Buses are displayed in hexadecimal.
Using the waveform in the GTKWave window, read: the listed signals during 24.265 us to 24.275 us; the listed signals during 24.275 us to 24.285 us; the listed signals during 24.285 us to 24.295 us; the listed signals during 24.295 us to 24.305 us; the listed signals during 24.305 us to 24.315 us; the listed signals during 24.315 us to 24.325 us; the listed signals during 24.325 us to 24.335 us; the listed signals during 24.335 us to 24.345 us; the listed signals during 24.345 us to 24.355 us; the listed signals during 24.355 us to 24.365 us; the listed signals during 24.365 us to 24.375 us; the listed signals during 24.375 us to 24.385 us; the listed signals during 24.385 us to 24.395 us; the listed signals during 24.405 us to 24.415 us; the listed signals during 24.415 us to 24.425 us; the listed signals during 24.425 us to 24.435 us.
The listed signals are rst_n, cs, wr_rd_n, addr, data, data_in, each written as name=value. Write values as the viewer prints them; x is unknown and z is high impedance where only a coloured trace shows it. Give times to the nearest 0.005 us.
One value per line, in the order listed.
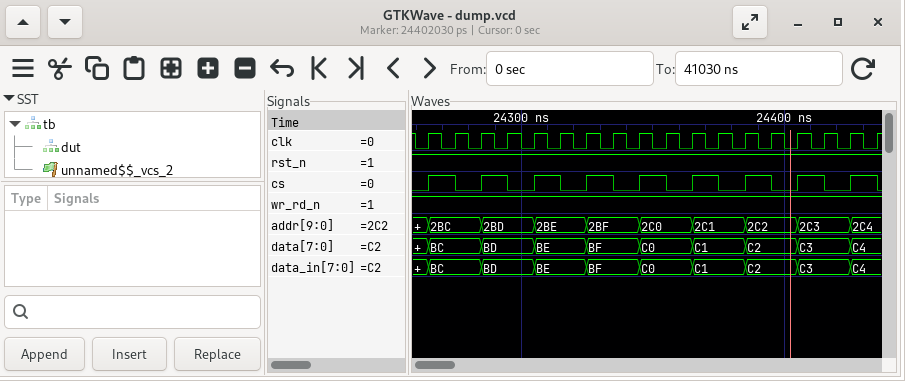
rst_n=1, cs=1, wr_rd_n=1, addr=2BC, data=BC, data_in=BC
rst_n=1, cs=0, wr_rd_n=1, addr=2BC, data=BC, data_in=BC
rst_n=1, cs=1, wr_rd_n=1, addr=2BD, data=BD, data_in=BD
rst_n=1, cs=0, wr_rd_n=1, addr=2BD, data=BD, data_in=BD
rst_n=1, cs=1, wr_rd_n=1, addr=2BE, data=BE, data_in=BE
rst_n=1, cs=0, wr_rd_n=1, addr=2BE, data=BE, data_in=BE
rst_n=1, cs=1, wr_rd_n=1, addr=2BF, data=BF, data_in=BF
rst_n=1, cs=0, wr_rd_n=1, addr=2BF, data=BF, data_in=BF
rst_n=1, cs=1, wr_rd_n=1, addr=2C0, data=C0, data_in=C0
rst_n=1, cs=0, wr_rd_n=1, addr=2C0, data=C0, data_in=C0
rst_n=1, cs=1, wr_rd_n=1, addr=2C1, data=C1, data_in=C1
rst_n=1, cs=0, wr_rd_n=1, addr=2C1, data=C1, data_in=C1
rst_n=1, cs=1, wr_rd_n=1, addr=2C2, data=C2, data_in=C2
rst_n=1, cs=1, wr_rd_n=1, addr=2C3, data=C3, data_in=C3
rst_n=1, cs=0, wr_rd_n=1, addr=2C3, data=C3, data_in=C3
rst_n=1, cs=1, wr_rd_n=1, addr=2C4, data=C4, data_in=C4
